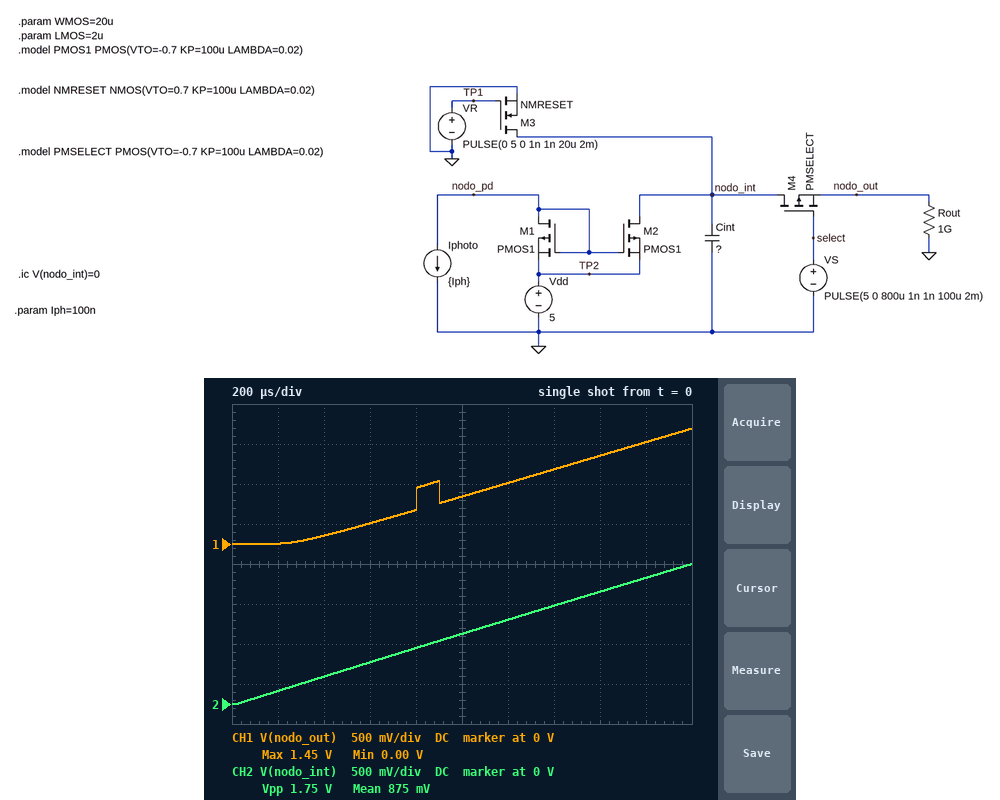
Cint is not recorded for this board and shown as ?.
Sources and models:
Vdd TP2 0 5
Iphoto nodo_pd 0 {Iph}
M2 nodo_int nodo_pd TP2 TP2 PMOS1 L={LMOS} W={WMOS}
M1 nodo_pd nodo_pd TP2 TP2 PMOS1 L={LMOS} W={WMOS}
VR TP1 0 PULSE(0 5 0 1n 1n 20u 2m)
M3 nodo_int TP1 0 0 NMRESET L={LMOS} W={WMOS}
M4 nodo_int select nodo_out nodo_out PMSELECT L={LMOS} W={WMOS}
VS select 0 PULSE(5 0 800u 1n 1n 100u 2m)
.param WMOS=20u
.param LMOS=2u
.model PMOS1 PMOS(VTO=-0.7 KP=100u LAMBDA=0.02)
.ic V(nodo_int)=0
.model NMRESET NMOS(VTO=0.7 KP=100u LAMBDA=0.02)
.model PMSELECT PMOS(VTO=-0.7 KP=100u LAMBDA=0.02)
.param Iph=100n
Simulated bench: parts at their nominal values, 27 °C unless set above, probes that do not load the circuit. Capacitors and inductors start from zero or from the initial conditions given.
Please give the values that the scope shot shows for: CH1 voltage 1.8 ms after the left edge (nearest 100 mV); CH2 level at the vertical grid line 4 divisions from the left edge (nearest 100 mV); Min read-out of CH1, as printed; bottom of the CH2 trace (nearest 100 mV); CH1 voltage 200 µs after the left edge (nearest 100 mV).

1.3 V
700 mV
0.00 V
0 V
0 V
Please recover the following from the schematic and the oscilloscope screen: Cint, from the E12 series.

120 pF
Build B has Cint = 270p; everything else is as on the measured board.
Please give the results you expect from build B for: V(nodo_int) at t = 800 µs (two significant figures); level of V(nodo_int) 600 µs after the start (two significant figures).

310 mV
230 mV
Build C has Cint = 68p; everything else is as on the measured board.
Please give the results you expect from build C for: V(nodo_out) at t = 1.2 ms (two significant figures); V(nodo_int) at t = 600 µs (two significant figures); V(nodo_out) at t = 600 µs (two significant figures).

1.5 V
920 mV
630 mV
